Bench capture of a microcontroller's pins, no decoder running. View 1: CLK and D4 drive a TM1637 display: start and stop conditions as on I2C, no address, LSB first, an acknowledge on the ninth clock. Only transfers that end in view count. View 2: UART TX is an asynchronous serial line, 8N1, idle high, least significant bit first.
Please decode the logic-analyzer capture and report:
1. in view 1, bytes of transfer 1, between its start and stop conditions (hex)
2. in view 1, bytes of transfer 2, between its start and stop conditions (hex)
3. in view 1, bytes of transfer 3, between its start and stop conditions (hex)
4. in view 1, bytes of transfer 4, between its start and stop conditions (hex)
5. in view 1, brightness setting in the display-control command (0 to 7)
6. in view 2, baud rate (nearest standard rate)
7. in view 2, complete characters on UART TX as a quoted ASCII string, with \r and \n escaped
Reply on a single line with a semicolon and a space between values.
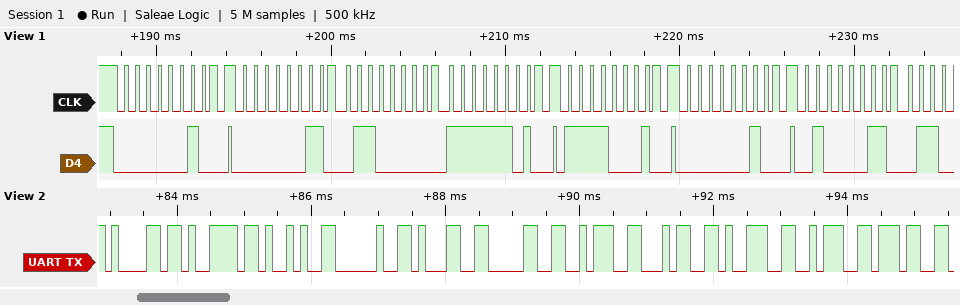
40; C0 06 BF; 8F; 40; 7; 9600 baud; "ay) 10:49:7"
